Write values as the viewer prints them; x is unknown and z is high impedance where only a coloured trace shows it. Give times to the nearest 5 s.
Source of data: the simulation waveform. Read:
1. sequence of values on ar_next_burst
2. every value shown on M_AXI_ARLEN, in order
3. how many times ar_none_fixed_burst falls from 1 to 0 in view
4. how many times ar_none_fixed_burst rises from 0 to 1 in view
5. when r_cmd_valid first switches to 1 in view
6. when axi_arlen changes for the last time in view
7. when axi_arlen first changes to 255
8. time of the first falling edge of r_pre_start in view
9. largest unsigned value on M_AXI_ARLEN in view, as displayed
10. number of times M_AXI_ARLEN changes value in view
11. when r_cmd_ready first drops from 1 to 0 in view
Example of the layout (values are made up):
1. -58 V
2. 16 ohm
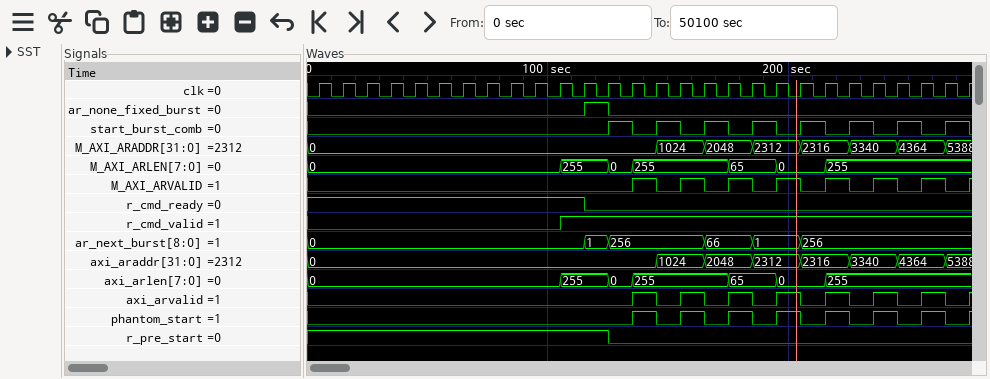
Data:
1. 0, 1, 256, 66, 1, 256
2. 0, 255, 0, 255, 65, 0, 255
3. 1
4. 1
5. 105 s
6. 215 s
7. 105 s
8. 125 s
9. 255
10. 6
11. 115 s
